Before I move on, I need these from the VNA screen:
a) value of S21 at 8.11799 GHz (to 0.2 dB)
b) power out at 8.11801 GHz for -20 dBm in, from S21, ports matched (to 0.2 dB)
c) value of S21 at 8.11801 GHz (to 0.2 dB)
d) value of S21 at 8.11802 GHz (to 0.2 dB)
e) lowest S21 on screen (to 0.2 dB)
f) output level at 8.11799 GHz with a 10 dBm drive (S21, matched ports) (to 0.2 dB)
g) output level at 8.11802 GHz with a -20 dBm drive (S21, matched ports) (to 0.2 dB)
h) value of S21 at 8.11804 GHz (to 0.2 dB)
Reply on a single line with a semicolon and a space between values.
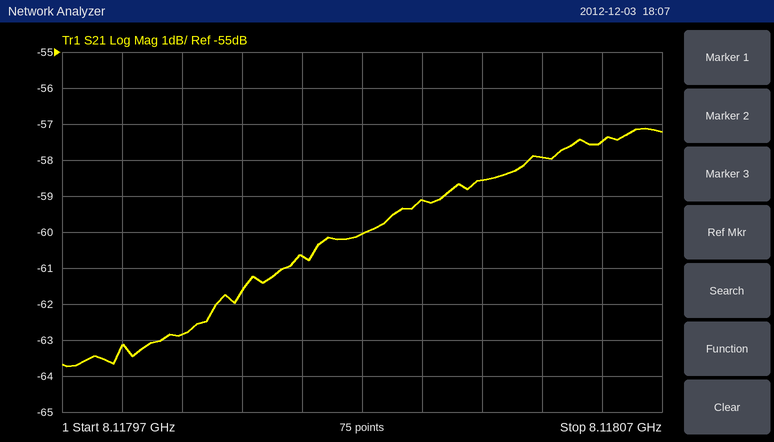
-62.8 dB; -80.6 dBm; -60.6 dB; -60.0 dB; -63.8 dB; -52.8 dBm; -80.0 dBm; -58.6 dB
